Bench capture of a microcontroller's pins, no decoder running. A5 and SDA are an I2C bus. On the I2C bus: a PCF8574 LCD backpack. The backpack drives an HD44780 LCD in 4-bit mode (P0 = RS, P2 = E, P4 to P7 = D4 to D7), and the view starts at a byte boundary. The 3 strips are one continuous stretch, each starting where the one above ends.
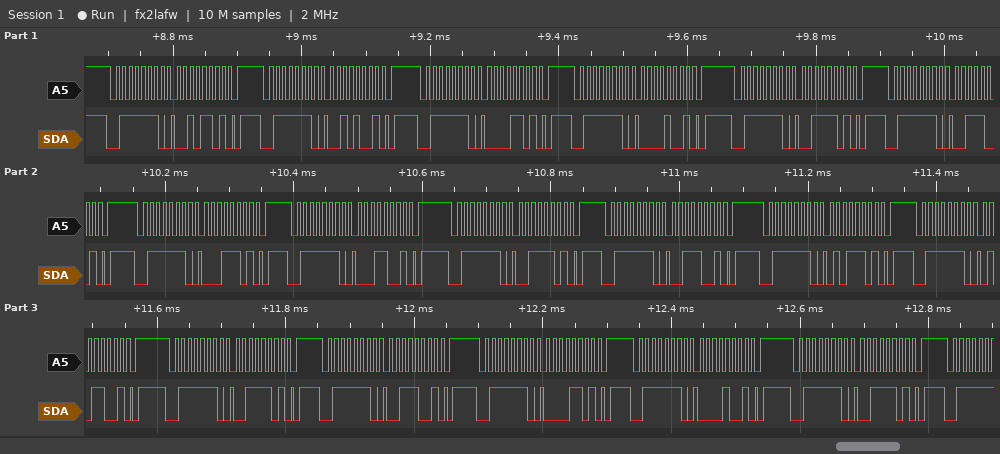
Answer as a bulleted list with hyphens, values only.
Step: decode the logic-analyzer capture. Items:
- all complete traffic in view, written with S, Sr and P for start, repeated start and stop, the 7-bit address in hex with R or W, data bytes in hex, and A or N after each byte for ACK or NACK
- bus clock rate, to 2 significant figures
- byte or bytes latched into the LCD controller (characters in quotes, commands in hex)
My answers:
- S 3FW A 2D A P S 3FW A 29 A P S 3FW A 0D A P S 3FW A 09 A P S 3FW A 3D A P S 3FW A 39 A P S 3FW A 1D A P S 3FW A 19 A P S 3FW A 3D A P S 3FW A 39 A P S 3FW A 5D A P S 3FW A 59 A P S 3FW A 3D A P S 3FW A 39 A P S 3FW A 0D A P S 3FW A 09 A P S 3FW A 3D A P
- 100 kHz
- ' ' '1' '5' '0'
